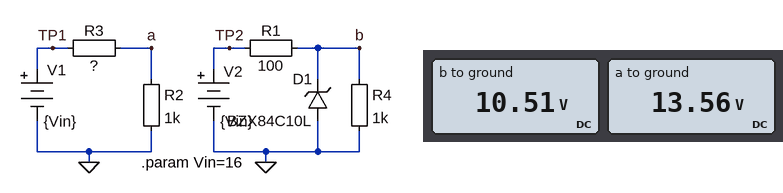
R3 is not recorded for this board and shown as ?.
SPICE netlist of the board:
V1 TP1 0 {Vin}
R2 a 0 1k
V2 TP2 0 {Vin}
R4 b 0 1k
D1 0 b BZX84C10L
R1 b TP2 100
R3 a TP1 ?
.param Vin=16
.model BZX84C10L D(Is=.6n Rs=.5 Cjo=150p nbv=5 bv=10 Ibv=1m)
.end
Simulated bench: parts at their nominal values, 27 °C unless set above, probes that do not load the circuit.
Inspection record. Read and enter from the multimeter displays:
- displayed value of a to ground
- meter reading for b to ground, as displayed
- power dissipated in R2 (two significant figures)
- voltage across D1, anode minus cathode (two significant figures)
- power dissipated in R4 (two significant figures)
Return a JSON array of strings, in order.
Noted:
["13.56 V", "10.51 V", "180 mW", "-11 V", "110 mW"]
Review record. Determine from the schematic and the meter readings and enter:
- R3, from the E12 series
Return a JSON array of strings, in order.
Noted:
["180 Ω"]
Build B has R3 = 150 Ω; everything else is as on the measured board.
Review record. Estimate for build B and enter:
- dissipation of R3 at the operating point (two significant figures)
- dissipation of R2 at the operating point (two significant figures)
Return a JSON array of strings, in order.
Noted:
["29 mW", "190 mW"]
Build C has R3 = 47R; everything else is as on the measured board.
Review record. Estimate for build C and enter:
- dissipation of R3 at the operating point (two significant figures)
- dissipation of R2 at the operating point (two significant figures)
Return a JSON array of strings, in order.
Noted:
["11 mW", "230 mW"]
